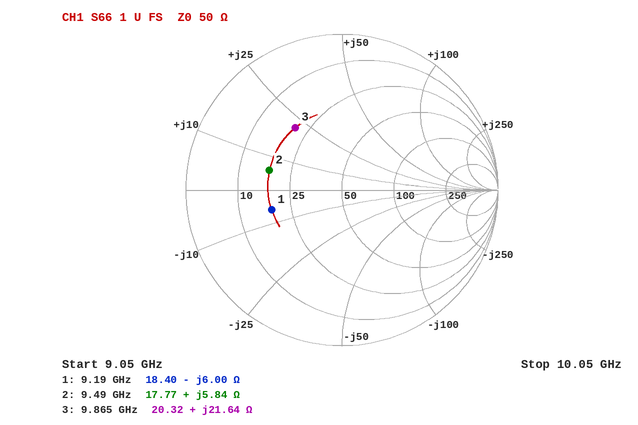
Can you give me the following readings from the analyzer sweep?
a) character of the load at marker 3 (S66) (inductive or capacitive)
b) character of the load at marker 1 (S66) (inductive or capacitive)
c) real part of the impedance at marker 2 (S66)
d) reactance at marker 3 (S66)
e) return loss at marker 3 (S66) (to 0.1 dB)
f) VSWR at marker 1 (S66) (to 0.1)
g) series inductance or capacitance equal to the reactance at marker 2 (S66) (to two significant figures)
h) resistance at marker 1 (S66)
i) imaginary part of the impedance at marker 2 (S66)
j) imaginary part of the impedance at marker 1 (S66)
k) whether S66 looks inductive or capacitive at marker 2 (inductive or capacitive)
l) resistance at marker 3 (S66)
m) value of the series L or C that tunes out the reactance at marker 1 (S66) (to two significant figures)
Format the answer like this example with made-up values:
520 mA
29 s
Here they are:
inductive
capacitive
17.77 Ω
+21.64 Ω
6.0 dB
2.8
98 pH
18.40 Ω
+5.84 Ω
-6.00 Ω
inductive
20.32 Ω
100 pH
